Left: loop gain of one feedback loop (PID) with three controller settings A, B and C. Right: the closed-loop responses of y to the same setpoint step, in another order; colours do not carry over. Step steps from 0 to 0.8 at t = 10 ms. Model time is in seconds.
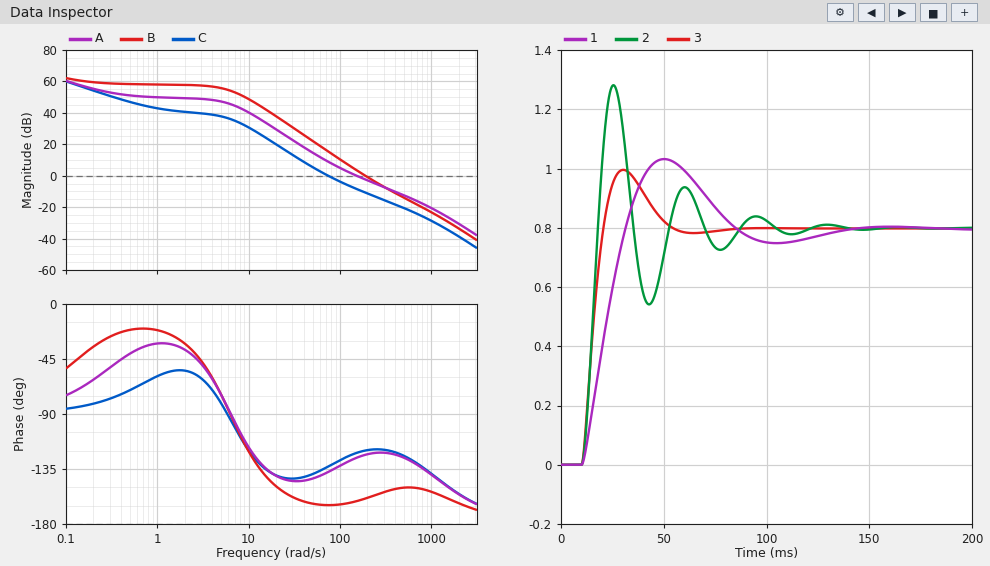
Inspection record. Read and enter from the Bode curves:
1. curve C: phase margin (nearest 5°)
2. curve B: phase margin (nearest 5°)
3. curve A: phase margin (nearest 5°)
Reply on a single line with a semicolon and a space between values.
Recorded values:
45°; 20°; 55°
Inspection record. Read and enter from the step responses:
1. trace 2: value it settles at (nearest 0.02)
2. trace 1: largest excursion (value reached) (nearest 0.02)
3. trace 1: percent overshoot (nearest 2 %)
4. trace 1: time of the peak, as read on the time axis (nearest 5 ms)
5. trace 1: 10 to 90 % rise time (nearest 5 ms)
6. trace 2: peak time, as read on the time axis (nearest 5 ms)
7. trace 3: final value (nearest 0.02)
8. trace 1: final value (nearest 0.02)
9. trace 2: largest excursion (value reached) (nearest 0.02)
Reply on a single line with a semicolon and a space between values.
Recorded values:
0.80; 1.04; 30 %; 50 ms; 15 ms; 25 ms; 0.80; 0.80; 1.28
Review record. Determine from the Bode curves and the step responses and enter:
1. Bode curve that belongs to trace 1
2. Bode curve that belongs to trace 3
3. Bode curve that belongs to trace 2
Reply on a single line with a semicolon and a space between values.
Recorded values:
C; A; B
